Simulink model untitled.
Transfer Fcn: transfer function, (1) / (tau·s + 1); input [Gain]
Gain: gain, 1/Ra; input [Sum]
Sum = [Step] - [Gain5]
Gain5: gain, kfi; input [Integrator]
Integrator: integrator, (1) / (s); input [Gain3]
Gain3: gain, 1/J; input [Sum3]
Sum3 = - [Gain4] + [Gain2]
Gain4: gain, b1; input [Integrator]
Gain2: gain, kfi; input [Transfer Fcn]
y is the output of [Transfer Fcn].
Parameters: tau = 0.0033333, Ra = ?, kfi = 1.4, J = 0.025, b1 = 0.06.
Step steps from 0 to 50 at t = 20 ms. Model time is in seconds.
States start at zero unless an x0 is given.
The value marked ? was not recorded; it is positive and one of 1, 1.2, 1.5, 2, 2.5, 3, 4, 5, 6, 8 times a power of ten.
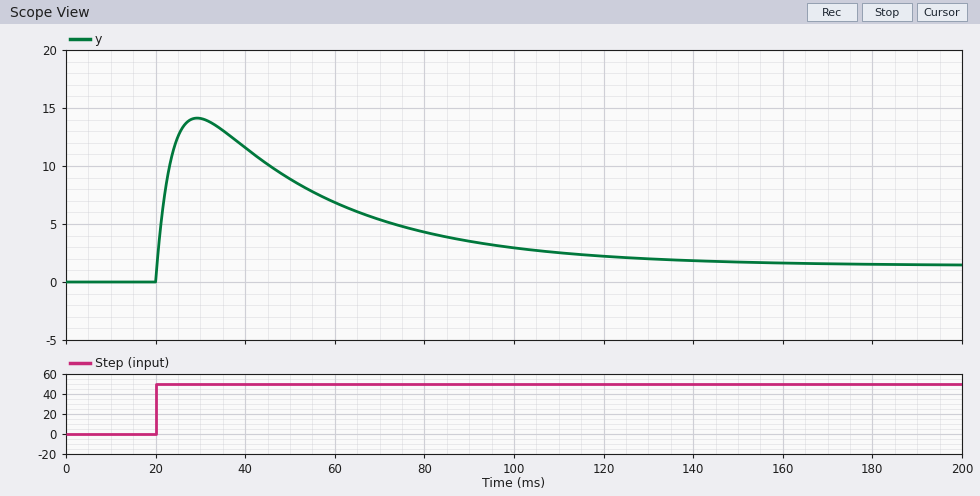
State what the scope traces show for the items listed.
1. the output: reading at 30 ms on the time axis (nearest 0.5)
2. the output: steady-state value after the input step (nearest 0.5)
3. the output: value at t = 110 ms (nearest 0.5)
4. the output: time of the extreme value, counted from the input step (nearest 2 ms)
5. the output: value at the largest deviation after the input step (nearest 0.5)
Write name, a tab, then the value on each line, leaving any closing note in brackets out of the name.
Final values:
the output: reading at 30 ms on the time axis	14.0
the output: steady-state value after the input step	1.5
the output: value at t = 110 ms	2.5
the output: time of the extreme value, counted from the input step	10 ms
the output: value at the largest deviation after the input step	14.0
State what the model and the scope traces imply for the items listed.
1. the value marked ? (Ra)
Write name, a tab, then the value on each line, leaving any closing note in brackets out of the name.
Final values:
the value marked ?	3
